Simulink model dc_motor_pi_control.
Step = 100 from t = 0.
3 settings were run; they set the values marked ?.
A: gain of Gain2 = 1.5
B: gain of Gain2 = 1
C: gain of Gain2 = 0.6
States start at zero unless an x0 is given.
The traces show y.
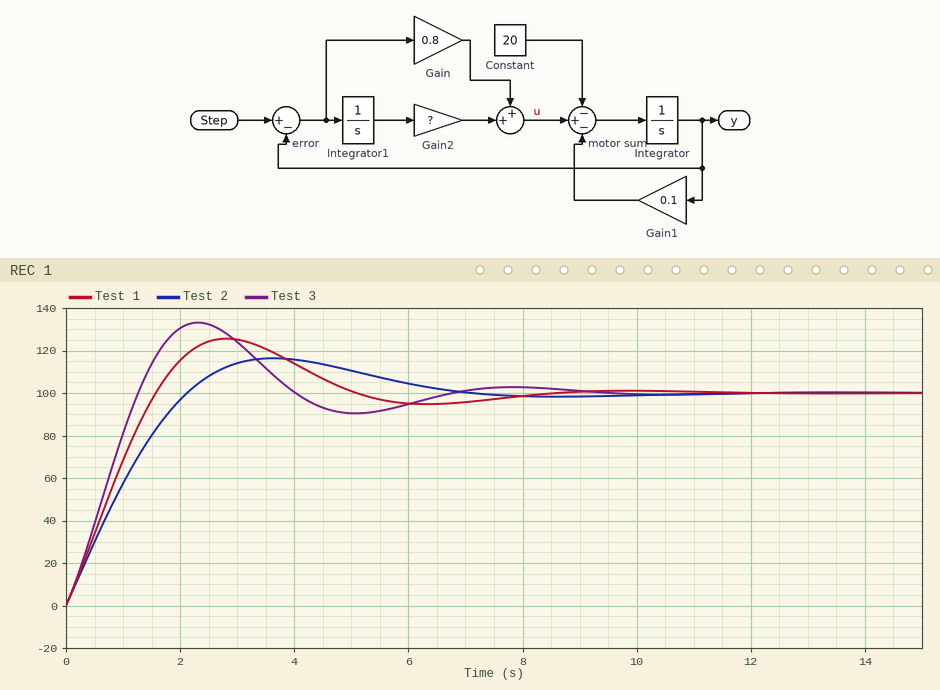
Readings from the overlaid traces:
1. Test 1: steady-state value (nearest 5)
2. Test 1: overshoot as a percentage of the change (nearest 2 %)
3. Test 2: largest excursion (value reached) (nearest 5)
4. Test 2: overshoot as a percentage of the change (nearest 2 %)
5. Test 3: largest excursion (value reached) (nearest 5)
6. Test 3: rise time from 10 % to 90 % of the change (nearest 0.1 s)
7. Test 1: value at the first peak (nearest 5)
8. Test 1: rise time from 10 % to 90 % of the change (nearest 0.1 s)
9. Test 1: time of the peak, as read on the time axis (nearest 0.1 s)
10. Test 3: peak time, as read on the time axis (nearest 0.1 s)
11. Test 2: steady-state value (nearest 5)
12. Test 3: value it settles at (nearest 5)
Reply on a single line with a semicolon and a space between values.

100; 26 %; 115; 16 %; 135; 1.0 s; 125; 1.2 s; 2.8 s; 2.3 s; 100; 100
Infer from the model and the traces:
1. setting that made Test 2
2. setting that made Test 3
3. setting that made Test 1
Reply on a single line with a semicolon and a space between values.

C; A; B
